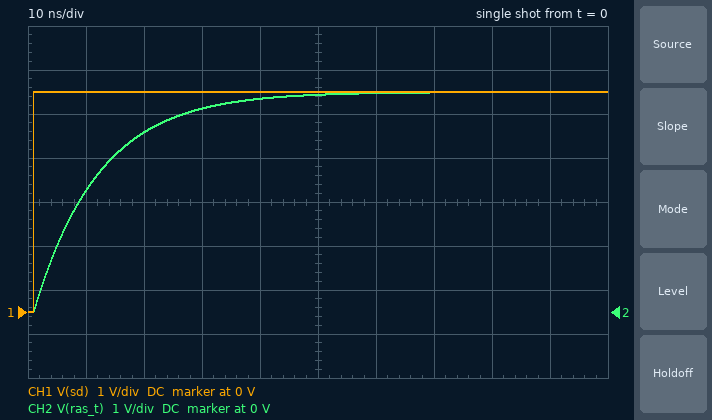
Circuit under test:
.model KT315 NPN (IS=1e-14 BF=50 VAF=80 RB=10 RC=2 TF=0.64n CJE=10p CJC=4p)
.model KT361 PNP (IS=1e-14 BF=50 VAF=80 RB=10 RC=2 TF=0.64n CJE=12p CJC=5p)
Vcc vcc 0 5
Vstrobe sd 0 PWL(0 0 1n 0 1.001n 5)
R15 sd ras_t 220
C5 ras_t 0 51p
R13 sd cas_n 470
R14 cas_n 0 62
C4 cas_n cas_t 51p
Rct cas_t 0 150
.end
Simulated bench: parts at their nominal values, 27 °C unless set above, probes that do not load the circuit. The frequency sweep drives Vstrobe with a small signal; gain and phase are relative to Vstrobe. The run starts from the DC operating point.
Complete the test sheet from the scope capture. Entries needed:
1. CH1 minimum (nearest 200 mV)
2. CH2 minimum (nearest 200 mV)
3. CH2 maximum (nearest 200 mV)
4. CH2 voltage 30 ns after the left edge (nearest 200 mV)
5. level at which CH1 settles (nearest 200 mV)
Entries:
0 V
0 V
5.0 V
4.6 V
5.0 V
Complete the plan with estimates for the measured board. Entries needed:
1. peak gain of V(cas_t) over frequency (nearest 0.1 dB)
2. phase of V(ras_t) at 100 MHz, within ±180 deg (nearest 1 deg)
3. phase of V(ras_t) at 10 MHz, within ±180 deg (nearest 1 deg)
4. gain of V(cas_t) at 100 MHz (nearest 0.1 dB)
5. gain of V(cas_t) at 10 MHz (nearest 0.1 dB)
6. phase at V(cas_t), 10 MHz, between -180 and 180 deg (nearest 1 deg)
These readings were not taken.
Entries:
-21.4 dB
-82 deg
-35 deg
-21.5 dB
-26.6 dB
57 deg
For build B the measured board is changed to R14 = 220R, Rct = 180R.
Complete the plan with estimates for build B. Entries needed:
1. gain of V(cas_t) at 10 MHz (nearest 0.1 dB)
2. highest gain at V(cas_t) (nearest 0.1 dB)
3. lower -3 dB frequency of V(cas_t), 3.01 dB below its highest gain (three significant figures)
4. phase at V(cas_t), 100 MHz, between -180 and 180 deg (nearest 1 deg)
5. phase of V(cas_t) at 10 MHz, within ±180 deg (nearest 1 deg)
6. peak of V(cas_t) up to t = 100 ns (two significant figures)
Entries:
-18.0 dB
-15.2 dB
9.46 MHz
5 deg
43 deg
870 mV
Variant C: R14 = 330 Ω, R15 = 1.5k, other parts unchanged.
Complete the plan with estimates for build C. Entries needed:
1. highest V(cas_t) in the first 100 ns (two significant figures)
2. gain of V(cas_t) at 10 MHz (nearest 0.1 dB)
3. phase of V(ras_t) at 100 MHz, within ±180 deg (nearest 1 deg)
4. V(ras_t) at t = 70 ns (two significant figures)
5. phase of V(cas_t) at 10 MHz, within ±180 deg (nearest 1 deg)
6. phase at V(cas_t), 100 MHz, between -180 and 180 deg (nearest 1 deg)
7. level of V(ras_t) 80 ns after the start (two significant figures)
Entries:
900 mV
-17.5 dB
-89 deg
3.0 V
42 deg
5 deg
3.2 V
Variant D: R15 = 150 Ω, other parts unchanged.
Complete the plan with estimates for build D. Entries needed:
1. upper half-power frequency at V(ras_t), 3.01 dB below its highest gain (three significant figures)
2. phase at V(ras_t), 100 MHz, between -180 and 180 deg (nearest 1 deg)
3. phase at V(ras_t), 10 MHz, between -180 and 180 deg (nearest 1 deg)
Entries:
20.8 MHz
-78 deg
-26 deg
